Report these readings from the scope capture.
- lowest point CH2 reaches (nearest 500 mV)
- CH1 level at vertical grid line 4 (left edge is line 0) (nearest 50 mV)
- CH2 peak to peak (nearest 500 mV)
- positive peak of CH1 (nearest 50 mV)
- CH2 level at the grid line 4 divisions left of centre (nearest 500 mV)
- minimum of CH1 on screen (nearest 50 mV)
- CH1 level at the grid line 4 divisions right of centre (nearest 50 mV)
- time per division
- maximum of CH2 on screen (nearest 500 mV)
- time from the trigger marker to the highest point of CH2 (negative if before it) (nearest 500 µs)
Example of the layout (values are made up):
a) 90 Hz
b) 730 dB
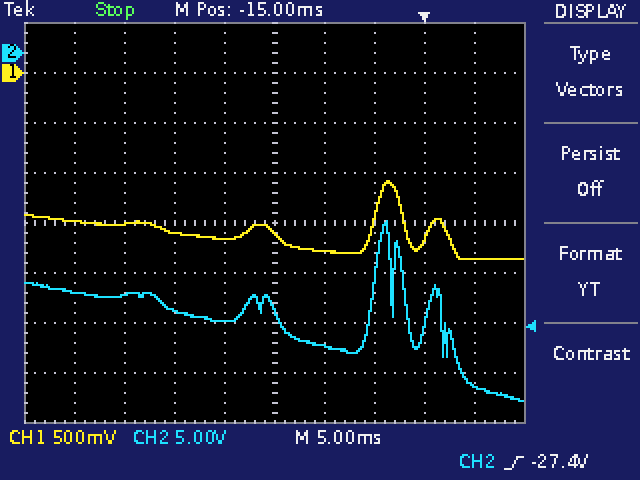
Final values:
a) -35.0 V
b) -1.65 V
c) 18.0 V
d) -1.10 V
e) -24.0 V
f) -1.85 V
g) -1.85 V
h) 5 ms
i) -17.0 V
j) -4.0 ms
